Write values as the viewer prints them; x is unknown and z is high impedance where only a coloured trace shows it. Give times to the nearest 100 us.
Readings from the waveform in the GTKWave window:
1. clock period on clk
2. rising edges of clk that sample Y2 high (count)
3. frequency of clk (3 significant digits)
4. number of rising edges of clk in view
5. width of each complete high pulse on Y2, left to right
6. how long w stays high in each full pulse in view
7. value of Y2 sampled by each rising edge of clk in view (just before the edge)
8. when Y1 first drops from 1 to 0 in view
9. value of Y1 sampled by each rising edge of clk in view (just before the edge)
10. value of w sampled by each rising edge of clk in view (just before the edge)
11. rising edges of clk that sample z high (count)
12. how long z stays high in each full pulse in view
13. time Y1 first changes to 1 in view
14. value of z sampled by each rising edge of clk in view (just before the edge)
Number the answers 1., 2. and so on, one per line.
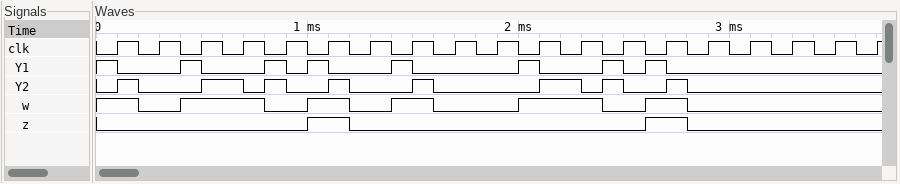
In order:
1. 200 us
2. 4
3. 5.00 kHz
4. 19
5. 100 us, 200 us, 100 us, 100 us, 100 us, 200 us, 100 us, 100 us
6. 400 us, 200 us, 200 us, 400 us, 200 us
7. 0 0 0 1 1 0 0 0 0 0 0 1 1 0 0 0 0 0 0
8. 100 us
9. 1 0 1 0 1 1 0 1 0 0 1 0 1 1 0 0 0 0 0
10. 1 0 1 1 0 1 0 1 0 0 1 1 0 1 0 0 0 0 0
11. 2
12. 200 us, 200 us
13. 400 us
14. 0 0 0 0 0 1 0 0 0 0 0 0 0 1 0 0 0 0 0
